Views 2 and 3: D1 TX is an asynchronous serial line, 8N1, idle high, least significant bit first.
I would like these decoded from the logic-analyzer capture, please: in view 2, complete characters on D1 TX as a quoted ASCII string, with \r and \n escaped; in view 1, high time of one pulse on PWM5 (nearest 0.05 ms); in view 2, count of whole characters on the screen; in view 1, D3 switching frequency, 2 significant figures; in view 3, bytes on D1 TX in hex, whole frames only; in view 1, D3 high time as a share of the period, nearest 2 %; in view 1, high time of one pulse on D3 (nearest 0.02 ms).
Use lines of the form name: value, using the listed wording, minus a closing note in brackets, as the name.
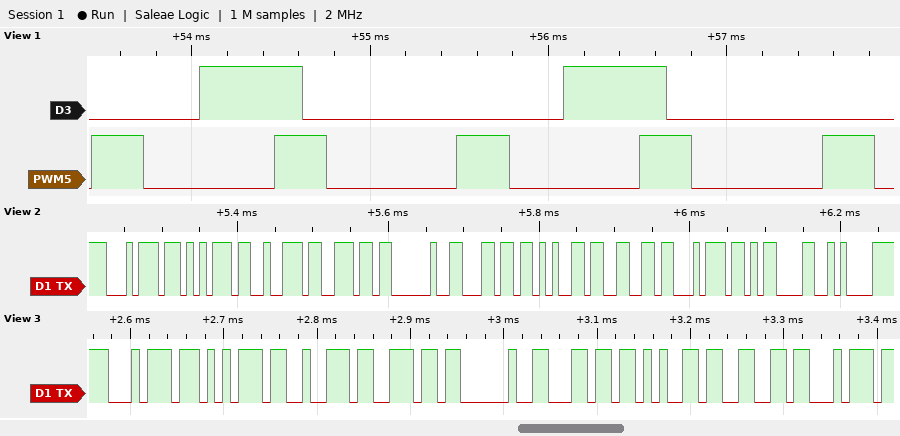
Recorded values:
in view 2, complete characters on D1 TX as a quoted ASCII string, with \r and \n escaped: "turn left\r\n"
in view 1, high time of one pulse on PWM5: 0.30 ms
in view 2, count of whole characters on the screen: 11
in view 1, D3 switching frequency, 2 significant figures: 490 Hz
in view 3, bytes on D1 TX in hex, whole frames only: 74 75 72 6E 20 6C 65 66 74
in view 1, D3 high time as a share of the period, nearest 2 %: 28 %
in view 1, high time of one pulse on D3: 0.58 ms
